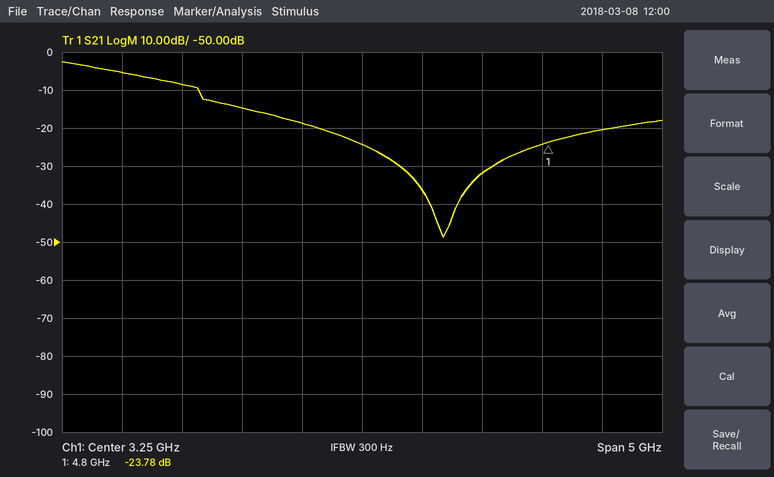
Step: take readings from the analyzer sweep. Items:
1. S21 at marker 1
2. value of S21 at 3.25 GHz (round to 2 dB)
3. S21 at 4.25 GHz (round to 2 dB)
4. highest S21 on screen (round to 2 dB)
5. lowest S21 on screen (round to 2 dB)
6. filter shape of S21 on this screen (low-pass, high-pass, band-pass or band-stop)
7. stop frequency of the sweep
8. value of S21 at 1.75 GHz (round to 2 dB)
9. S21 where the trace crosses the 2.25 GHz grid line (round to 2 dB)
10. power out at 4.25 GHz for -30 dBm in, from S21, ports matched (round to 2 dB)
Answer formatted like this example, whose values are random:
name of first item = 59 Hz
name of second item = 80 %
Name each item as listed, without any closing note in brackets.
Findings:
S21 at marker 1 = -23.78 dB
value of S21 at 3.25 GHz = -24 dB
S21 at 4.25 GHz = -32 dB
highest S21 on screen = -2 dB
lowest S21 on screen = -48 dB
filter shape of S21 on this screen = low-pass
stop frequency of the sweep = 5.75 GHz
value of S21 at 1.75 GHz = -8 dB
S21 where the trace crosses the 2.25 GHz grid line = -14 dB
power out at 4.25 GHz for -30 dBm in, from S21, ports matched = -62 dBm
